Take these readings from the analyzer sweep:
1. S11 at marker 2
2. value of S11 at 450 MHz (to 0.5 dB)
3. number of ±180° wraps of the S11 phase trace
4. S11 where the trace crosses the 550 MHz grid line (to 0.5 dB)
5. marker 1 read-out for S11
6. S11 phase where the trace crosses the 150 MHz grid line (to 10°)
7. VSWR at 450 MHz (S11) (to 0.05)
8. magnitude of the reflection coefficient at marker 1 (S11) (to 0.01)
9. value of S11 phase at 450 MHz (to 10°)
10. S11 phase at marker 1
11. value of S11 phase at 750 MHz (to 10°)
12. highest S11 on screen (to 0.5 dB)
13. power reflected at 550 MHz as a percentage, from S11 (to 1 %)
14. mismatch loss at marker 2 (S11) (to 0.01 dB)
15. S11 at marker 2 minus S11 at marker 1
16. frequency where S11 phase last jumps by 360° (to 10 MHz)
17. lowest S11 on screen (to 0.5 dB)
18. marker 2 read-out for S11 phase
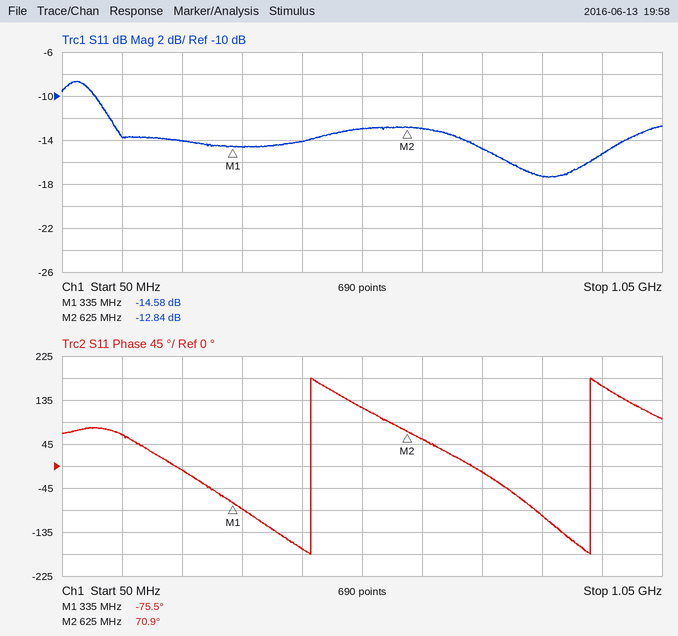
-12.84 dB
-14.0 dB
2
-13.0 dB
-14.58 dB
60°
1.50
0.19
-170°
-75.5°
-10°
-8.5 dB
5 %
0.23 dB
1.74 dB
930 MHz
-17.5 dB
70.9°
